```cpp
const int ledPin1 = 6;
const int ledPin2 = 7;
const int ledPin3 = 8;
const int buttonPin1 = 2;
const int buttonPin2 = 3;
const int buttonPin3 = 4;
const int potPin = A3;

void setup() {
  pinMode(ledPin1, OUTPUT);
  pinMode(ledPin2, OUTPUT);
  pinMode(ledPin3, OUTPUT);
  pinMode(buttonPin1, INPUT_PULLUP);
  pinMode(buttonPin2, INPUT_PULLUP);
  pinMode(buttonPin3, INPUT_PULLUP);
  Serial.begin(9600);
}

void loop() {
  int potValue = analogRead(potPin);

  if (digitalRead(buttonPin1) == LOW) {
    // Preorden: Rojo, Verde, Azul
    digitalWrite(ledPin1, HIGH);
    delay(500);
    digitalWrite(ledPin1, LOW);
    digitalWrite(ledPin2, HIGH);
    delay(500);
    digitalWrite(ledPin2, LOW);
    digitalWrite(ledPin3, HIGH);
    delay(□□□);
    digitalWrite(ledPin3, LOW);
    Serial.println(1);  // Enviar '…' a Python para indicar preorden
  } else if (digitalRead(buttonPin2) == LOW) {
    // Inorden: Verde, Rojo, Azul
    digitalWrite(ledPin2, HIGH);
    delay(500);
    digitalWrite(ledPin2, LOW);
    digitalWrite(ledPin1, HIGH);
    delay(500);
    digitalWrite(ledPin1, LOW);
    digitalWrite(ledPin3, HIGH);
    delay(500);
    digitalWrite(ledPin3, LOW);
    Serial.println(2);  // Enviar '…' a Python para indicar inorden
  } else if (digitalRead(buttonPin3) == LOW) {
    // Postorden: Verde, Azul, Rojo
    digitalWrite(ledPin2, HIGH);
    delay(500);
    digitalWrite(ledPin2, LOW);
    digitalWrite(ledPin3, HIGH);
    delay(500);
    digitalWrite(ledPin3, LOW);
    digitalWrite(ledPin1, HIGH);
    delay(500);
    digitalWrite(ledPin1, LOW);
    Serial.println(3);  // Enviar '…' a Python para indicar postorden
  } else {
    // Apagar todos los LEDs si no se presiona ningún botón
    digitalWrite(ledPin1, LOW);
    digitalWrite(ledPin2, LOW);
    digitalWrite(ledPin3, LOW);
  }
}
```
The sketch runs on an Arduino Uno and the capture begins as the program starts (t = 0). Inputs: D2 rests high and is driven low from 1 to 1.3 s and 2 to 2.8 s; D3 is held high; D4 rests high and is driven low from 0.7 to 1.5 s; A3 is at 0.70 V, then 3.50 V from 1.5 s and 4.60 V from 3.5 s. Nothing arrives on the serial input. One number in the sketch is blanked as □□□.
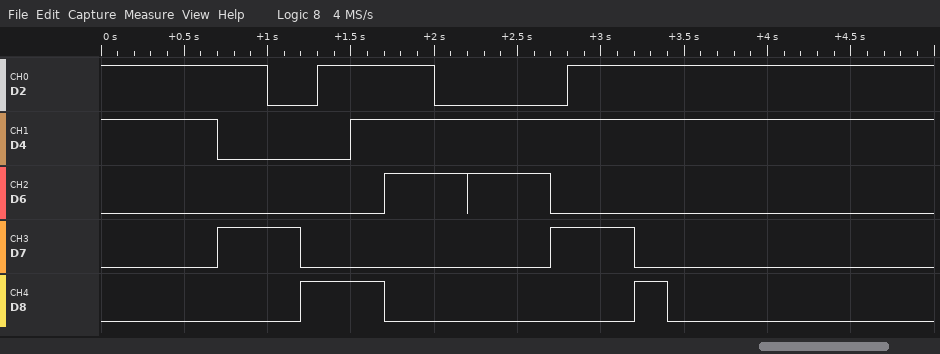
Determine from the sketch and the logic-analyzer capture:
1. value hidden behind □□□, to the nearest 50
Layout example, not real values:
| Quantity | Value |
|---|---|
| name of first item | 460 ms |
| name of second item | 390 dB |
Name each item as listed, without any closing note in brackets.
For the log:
| Quantity | Value |
|---|---|
| value hidden behind □□□, to the nearest 50 | 200 |
